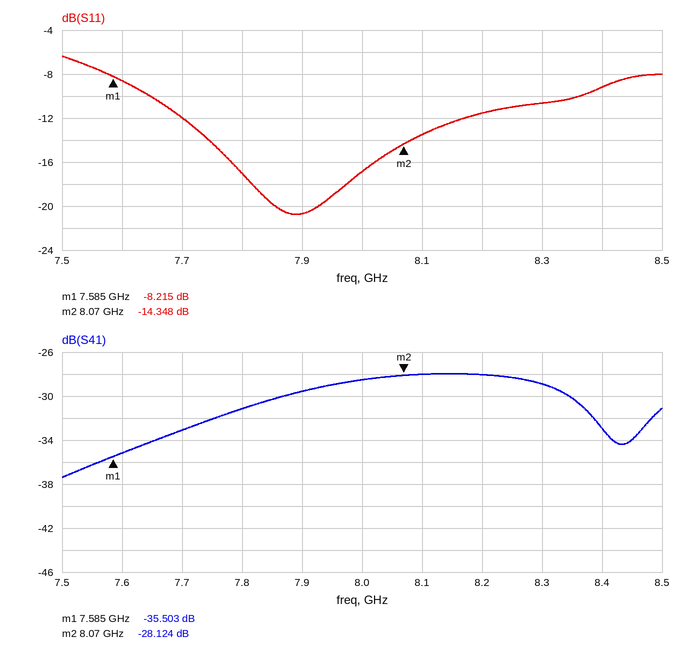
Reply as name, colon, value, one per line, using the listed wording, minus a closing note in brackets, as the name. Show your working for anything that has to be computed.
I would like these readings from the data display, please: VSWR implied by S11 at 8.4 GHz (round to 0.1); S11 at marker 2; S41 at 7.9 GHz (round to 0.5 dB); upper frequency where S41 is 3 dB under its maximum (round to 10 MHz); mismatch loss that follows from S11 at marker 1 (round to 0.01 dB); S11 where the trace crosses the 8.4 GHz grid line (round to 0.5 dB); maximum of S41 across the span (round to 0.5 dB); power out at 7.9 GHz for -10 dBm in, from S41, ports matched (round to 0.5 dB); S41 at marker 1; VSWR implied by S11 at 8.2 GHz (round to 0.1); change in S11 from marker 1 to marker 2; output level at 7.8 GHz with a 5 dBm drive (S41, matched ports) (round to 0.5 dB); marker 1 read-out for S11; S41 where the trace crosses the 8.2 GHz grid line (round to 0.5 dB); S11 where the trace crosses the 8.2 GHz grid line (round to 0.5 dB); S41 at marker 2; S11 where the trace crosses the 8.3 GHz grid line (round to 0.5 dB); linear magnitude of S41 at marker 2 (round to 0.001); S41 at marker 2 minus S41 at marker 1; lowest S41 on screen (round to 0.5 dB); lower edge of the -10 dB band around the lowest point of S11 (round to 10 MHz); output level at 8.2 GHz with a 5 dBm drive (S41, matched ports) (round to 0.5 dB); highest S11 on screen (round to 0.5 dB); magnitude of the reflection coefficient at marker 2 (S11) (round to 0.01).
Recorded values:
VSWR implied by S11 at 8.4 GHz: |Γ| = 10^(-9/20) = 0.3548; VSWR = (1 + 0.3548)/(1 − 0.3548) ≈ 2.1
S11 at marker 2: -14.348 dB
S41 at 7.9 GHz: -29.5 dB
upper frequency where S41 is 3 dB under its maximum: 8.37 GHz
mismatch loss that follows from S11 at marker 1: −10 log10(1 − 10^(-8.215/10)) ≈ 0.71 dB
S11 where the trace crosses the 8.4 GHz grid line: -9.0 dB
maximum of S41 across the span: -28.0 dB
power out at 7.9 GHz for -10 dBm in, from S41, ports matched: -10 dBm + (-29.5 dB) = -39.5 dBm
S41 at marker 1: -35.503 dB
VSWR implied by S11 at 8.2 GHz: |Γ| = 10^(-11.5/20) = 0.2661; VSWR = (1 + 0.2661)/(1 − 0.2661) ≈ 1.7
change in S11 from marker 1 to marker 2: -14.348 − (-8.215) = -6.133 dB
output level at 7.8 GHz with a 5 dBm drive (S41, matched ports): 5 dBm + (-31.0 dB) = -26.0 dBm
marker 1 read-out for S11: -8.215 dB
S41 where the trace crosses the 8.2 GHz grid line: -28.0 dB
S11 where the trace crosses the 8.2 GHz grid line: -11.5 dB
S41 at marker 2: -28.124 dB
S11 where the trace crosses the 8.3 GHz grid line: -10.5 dB
linear magnitude of S41 at marker 2: 10^(-28.124/20) ≈ 0.039
S41 at marker 2 minus S41 at marker 1: -28.124 − (-35.503) = 7.379 dB
lowest S41 on screen: -37.5 dB
lower edge of the -10 dB band around the lowest point of S11: 7.65 GHz
output level at 8.2 GHz with a 5 dBm drive (S41, matched ports): 5 dBm + (-28.0 dB) = -23.0 dBm
highest S11 on screen: -6.5 dB
magnitude of the reflection coefficient at marker 2 (S11): 10^(-14.348/20) ≈ 0.19
